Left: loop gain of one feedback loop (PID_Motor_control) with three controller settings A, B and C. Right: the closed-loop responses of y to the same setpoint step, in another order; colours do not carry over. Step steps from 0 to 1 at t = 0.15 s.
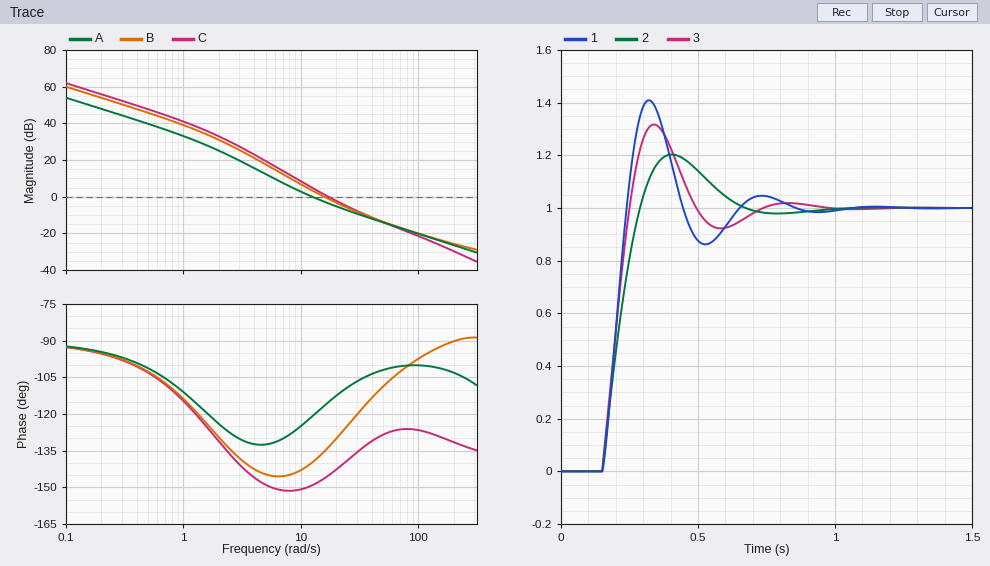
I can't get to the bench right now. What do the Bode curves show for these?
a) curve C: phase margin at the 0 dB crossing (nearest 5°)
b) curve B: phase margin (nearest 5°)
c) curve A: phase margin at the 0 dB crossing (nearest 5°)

35°
45°
60°
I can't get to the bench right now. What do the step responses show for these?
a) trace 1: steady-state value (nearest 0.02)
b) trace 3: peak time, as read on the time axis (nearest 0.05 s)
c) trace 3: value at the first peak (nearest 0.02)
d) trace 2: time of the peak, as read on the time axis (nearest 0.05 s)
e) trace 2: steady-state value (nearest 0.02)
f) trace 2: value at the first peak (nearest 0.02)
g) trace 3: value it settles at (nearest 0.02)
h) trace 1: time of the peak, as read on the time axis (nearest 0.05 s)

1.00
0.35 s
1.32
0.40 s
1.00
1.20
1.00
0.30 s
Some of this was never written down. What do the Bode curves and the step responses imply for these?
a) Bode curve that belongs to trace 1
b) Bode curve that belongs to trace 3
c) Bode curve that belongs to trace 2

C
B
A
